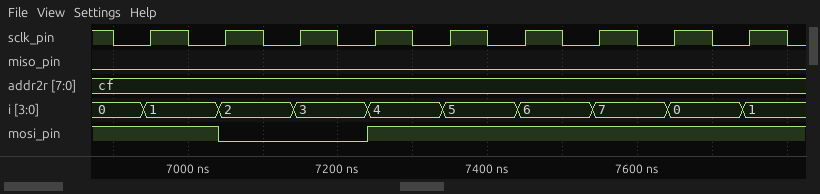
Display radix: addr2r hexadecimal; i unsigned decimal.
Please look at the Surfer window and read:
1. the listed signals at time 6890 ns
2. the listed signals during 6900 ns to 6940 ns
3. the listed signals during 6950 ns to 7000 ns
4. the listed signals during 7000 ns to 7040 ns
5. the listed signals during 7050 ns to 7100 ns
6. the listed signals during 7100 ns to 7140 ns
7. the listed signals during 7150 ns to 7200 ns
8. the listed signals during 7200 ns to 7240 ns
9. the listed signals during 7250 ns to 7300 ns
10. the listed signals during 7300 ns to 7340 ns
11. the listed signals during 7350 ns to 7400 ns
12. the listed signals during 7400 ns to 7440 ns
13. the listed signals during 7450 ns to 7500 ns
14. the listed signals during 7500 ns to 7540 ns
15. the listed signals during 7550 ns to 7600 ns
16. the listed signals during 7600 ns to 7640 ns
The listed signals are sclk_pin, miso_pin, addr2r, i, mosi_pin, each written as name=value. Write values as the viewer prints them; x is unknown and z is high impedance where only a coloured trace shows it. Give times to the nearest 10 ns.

sclk_pin=1, miso_pin=0, addr2r=cf, i=0, mosi_pin=1
sclk_pin=0, miso_pin=0, addr2r=cf, i=0, mosi_pin=1
sclk_pin=1, miso_pin=0, addr2r=cf, i=1, mosi_pin=1
sclk_pin=0, miso_pin=0, addr2r=cf, i=1, mosi_pin=1
sclk_pin=1, miso_pin=0, addr2r=cf, i=2, mosi_pin=0
sclk_pin=0, miso_pin=0, addr2r=cf, i=2, mosi_pin=0
sclk_pin=1, miso_pin=0, addr2r=cf, i=3, mosi_pin=0
sclk_pin=0, miso_pin=0, addr2r=cf, i=3, mosi_pin=0
sclk_pin=1, miso_pin=0, addr2r=cf, i=4, mosi_pin=1
sclk_pin=0, miso_pin=0, addr2r=cf, i=4, mosi_pin=1
sclk_pin=1, miso_pin=0, addr2r=cf, i=5, mosi_pin=1
sclk_pin=0, miso_pin=0, addr2r=cf, i=5, mosi_pin=1
sclk_pin=1, miso_pin=0, addr2r=cf, i=6, mosi_pin=1
sclk_pin=0, miso_pin=0, addr2r=cf, i=6, mosi_pin=1
sclk_pin=1, miso_pin=0, addr2r=cf, i=7, mosi_pin=1
sclk_pin=0, miso_pin=0, addr2r=cf, i=7, mosi_pin=1
